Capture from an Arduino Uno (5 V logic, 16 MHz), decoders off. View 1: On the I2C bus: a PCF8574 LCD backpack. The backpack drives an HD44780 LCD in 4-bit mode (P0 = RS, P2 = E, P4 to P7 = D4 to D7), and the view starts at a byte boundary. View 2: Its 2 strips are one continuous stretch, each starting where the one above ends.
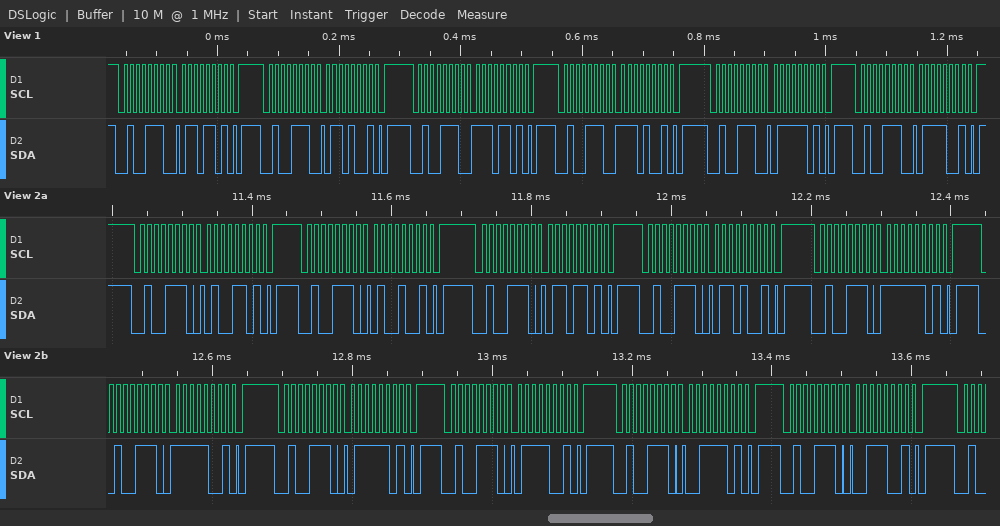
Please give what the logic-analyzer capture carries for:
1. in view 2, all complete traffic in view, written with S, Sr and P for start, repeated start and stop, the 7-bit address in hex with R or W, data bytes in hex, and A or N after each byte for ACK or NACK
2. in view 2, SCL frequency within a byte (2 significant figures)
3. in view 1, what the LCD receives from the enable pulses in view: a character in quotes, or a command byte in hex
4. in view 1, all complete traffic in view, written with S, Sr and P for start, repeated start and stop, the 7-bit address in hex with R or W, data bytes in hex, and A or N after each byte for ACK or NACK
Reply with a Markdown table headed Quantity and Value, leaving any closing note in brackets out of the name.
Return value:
| Quantity | Value |
|---|---|
| in view 2, all complete traffic in view, written with S, Sr and P for start, repeated start and stop, the 7-bit address in hex with R or W, data bytes in hex, and A or N after each byte for ACK or NACK | S 27W A 4D A P S 27W A 49 A P S 27W A 6D A P S 27W A 69 A P S 27W A FD A P S 27W A F9 A P S 27W A 7D A P S 27W A 79 A P S 27W A 3D A P S 27W A 39 A P |
| in view 2, SCL frequency within a byte | 100 kHz |
| in view 1, what the LCD receives from the enable pulses in view: a character in quotes, or a command byte in hex | 'n' |
| in view 1, all complete traffic in view, written with S, Sr and P for start, repeated start and stop, the 7-bit address in hex with R or W, data bytes in hex, and A or N after each byte for ACK or NACK | S 27W A 6D A P S 27W A 69 A P S 27W A ED A P S 27W A E9 A P S 27W A 7D A P S 27W A 79 A P |
